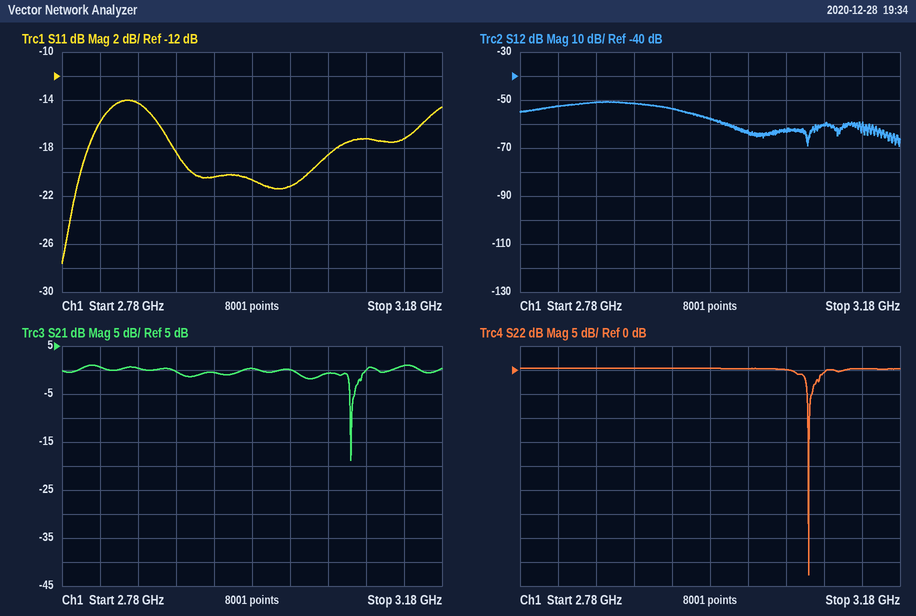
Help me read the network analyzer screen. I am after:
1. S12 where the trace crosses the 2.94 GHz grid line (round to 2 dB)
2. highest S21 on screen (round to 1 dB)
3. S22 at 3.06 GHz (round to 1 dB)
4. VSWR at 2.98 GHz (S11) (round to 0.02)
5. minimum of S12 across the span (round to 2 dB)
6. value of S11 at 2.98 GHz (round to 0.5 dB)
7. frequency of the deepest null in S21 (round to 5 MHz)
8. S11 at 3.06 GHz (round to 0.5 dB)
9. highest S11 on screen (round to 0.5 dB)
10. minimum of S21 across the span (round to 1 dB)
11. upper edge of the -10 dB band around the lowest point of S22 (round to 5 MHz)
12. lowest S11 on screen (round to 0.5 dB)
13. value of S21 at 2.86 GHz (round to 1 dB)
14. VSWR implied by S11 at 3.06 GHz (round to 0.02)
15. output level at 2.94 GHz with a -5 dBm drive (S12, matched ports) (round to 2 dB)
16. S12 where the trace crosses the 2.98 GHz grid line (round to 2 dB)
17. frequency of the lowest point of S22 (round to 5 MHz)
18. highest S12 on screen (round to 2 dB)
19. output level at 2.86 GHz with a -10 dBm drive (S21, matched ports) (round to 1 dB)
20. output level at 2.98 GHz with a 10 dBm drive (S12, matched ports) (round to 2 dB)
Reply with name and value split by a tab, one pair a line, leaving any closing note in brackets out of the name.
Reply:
S12 where the trace crosses the 2.94 GHz grid line	-54 dB
highest S21 on screen	1 dB
S22 at 3.06 GHz	0 dB
VSWR at 2.98 GHz (S11)	1.20
minimum of S12 across the span	-70 dB
value of S11 at 2.98 GHz	-20.5 dB
frequency of the deepest null in S21	3.085 GHz
S11 at 3.06 GHz	-18.5 dB
highest S11 on screen	-14.0 dB
minimum of S21 across the span	-19 dB
upper edge of the -10 dB band around the lowest point of S22	3.085 GHz
lowest S11 on screen	-27.5 dB
value of S21 at 2.86 GHz	0 dB
VSWR implied by S11 at 3.06 GHz	1.26
output level at 2.94 GHz with a -5 dBm drive (S12, matched ports)	-58 dBm
S12 where the trace crosses the 2.98 GHz grid line	-58 dB
frequency of the lowest point of S22	3.085 GHz
highest S12 on screen	-50 dB
output level at 2.86 GHz with a -10 dBm drive (S21, matched ports)	-10 dBm
output level at 2.98 GHz with a 10 dBm drive (S12, matched ports)	-48 dBm
